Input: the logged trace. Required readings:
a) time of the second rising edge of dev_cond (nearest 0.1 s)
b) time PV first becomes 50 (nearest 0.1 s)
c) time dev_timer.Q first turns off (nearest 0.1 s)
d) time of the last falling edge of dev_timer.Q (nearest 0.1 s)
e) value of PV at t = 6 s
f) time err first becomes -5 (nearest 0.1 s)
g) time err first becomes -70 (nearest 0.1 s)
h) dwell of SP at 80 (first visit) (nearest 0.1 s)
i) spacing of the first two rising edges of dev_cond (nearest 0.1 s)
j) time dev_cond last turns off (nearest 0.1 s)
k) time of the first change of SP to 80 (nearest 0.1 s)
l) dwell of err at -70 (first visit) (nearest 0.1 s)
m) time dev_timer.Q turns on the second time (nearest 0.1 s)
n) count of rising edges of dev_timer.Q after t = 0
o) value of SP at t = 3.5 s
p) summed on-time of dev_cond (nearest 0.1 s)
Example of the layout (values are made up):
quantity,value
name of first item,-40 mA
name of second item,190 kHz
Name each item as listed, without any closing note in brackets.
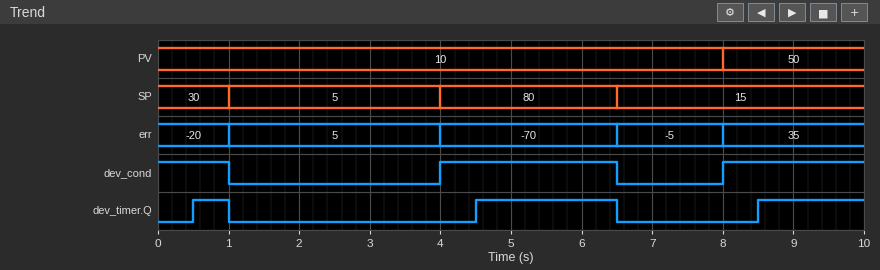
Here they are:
quantity,value
time of the second rising edge of dev_cond,8.0 s
time PV first becomes 50,8.0 s
time dev_timer.Q first turns off,1.0 s
time of the last falling edge of dev_timer.Q,6.5 s
value of PV at t = 6 s,10
time err first becomes -5,6.5 s
time err first becomes -70,4.0 s
dwell of SP at 80 (first visit),2.5 s
spacing of the first two rising edges of dev_cond,4.0 s
time dev_cond last turns off,6.5 s
time of the first change of SP to 80,4.0 s
dwell of err at -70 (first visit),2.5 s
time dev_timer.Q turns on the second time,4.5 s
count of rising edges of dev_timer.Q after t = 0,3
value of SP at t = 3.5 s,5
summed on-time of dev_cond,5.5 s
